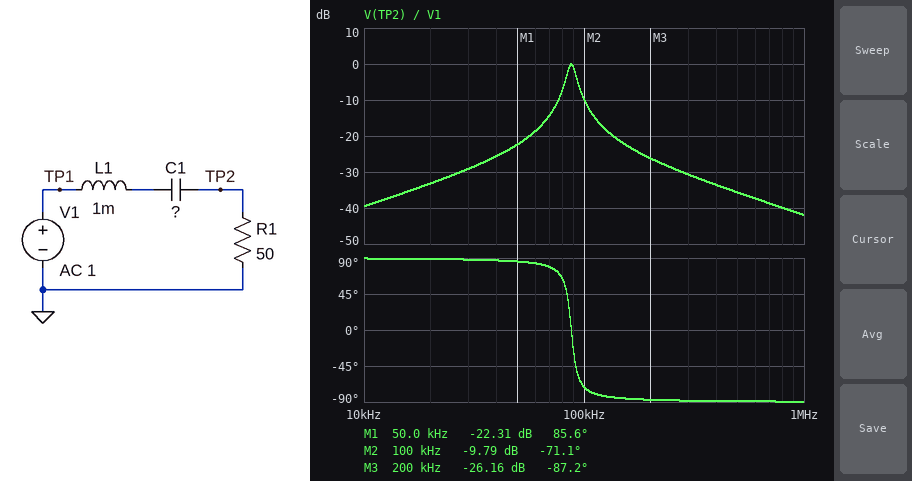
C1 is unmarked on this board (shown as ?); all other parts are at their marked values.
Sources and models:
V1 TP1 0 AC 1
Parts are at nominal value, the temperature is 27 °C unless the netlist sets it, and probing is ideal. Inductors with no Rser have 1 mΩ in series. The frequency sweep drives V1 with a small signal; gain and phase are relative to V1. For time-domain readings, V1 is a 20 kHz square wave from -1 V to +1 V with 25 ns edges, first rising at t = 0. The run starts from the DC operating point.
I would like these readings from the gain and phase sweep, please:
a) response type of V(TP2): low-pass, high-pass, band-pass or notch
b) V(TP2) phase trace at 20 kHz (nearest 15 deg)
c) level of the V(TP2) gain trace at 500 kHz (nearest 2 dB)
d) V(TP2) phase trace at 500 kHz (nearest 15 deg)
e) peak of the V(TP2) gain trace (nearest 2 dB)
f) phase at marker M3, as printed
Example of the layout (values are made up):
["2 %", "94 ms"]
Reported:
["band-pass", "90 deg", "-36 dB", "-90 deg", "0 dB", "-87.2 deg"]
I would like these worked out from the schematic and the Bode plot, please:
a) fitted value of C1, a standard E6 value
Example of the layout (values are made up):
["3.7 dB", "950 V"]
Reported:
["3.3 nF"]
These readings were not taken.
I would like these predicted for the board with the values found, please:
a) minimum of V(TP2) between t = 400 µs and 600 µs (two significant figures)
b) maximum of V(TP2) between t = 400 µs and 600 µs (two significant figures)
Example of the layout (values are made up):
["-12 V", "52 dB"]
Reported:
["-130 mV", "130 mV"]
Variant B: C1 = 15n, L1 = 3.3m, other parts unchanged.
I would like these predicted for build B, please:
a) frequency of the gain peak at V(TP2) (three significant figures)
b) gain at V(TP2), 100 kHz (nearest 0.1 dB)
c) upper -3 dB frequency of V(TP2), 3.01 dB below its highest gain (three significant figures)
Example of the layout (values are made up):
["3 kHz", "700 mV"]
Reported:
["22.6 kHz", "-31.9 dB", "23.9 kHz"]
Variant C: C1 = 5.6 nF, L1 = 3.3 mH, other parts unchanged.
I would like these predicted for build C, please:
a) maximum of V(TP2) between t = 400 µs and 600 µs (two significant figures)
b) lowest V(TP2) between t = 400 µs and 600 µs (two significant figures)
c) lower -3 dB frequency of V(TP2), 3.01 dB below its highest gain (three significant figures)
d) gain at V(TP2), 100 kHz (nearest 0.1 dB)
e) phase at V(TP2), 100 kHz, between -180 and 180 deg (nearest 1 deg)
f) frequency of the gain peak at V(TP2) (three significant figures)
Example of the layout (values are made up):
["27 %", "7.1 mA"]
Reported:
["70 mV", "-72 mV", "35.8 kHz", "-31.1 dB", "-88 deg", "37.0 kHz"]
